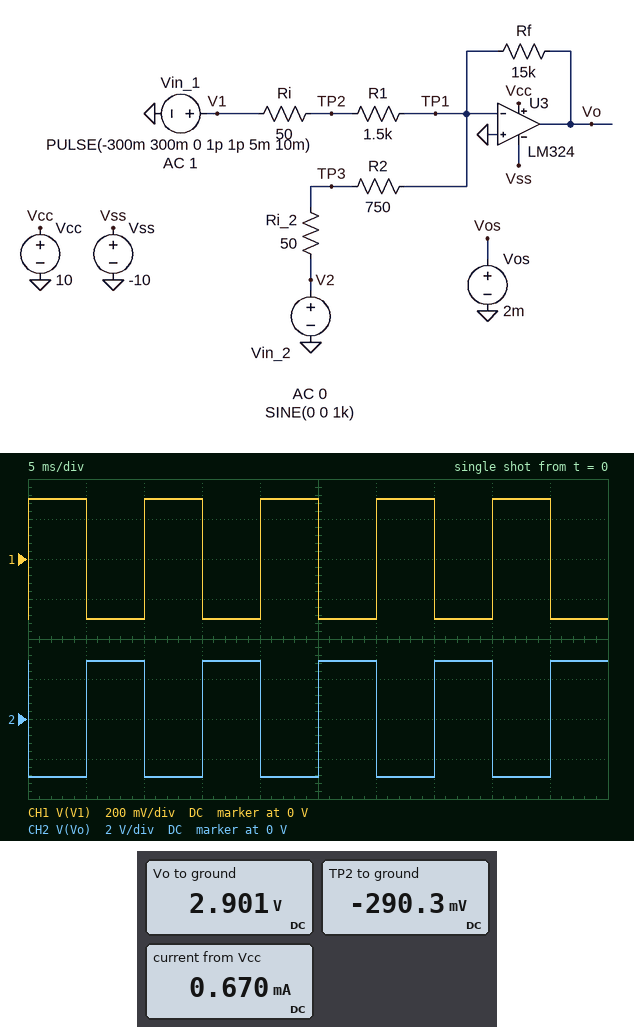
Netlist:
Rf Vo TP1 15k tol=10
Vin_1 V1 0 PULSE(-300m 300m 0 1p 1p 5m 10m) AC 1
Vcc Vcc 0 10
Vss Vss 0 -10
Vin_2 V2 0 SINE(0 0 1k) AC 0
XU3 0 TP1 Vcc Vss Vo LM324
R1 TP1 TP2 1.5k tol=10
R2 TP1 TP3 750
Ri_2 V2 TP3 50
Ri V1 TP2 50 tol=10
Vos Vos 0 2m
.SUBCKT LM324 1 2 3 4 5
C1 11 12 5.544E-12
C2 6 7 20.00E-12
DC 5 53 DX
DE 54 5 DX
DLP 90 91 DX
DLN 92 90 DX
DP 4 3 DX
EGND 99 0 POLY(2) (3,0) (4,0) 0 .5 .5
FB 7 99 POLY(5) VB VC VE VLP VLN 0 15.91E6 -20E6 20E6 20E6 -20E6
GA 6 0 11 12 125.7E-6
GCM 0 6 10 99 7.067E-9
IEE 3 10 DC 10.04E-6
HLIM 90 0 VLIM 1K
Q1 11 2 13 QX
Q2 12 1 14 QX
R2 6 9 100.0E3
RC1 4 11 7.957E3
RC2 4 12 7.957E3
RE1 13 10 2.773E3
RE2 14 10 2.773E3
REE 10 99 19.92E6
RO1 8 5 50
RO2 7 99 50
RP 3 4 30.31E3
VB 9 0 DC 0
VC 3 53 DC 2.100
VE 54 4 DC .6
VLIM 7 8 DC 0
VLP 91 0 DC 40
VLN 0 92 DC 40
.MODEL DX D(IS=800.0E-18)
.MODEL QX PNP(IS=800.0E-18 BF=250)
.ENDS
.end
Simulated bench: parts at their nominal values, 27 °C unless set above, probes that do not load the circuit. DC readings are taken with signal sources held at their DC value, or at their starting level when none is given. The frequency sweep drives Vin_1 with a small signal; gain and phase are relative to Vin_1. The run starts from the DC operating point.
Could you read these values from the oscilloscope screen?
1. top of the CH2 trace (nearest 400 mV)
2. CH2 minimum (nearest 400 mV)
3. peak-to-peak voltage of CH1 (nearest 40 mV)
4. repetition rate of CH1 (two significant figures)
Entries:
2.8 V
-2.8 V
600 mV
100 Hz
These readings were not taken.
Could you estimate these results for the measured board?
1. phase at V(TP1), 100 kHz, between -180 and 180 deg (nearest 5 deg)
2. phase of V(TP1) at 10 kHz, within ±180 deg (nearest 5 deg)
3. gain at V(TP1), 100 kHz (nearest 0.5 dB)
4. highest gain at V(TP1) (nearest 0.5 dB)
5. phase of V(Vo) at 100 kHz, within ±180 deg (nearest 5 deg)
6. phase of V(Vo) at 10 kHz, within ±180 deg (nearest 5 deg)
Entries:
20 deg
75 deg
-10.0 dB
-9.5 dB
105 deg
165 deg
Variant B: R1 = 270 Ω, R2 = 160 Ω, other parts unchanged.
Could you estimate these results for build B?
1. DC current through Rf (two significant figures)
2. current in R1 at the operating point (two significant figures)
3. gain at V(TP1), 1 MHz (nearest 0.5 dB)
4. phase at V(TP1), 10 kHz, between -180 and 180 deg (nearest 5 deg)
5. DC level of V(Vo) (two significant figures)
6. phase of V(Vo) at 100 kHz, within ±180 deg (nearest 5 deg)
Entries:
570 µA
790 µA
-8.0 dB
0 deg
8.5 V
125 deg
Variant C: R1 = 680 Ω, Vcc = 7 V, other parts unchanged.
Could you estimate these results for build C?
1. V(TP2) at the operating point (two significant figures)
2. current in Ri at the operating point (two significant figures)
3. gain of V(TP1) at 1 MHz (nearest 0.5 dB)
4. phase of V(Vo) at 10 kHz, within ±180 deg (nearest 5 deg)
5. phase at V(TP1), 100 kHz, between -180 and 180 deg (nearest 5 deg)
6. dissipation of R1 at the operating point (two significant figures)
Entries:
-280 mV
390 µA
-6.0 dB
170 deg
0 deg
100 µW
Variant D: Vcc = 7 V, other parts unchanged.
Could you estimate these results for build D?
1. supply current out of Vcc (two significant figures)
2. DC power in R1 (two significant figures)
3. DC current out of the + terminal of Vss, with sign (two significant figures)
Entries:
570 µA
56 µW
-570 µA
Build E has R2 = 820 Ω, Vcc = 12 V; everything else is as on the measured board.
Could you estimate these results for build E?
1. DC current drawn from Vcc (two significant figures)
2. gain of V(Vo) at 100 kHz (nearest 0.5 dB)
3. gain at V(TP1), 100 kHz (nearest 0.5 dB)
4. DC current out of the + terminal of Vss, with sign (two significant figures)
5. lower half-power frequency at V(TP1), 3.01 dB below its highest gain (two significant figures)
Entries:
740 µA
10.5 dB
-9.5 dB
-740 µA
36 kHz
